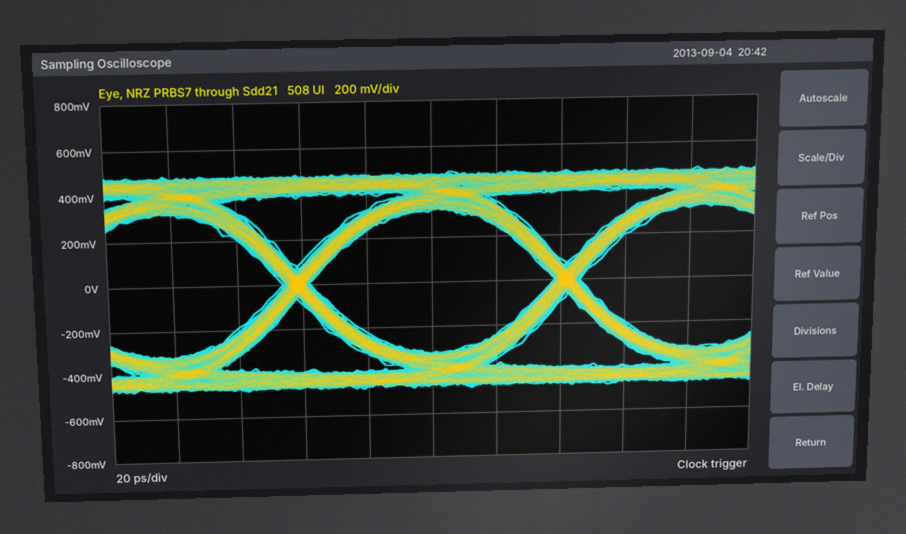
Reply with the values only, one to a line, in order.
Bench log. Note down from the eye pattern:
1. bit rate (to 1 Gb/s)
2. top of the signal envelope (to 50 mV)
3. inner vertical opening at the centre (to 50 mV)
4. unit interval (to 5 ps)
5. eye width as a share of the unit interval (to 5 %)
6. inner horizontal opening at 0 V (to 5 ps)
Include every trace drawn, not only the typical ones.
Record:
12 Gb/s
500 mV
650 mV
85 ps
90 %
75 ps
